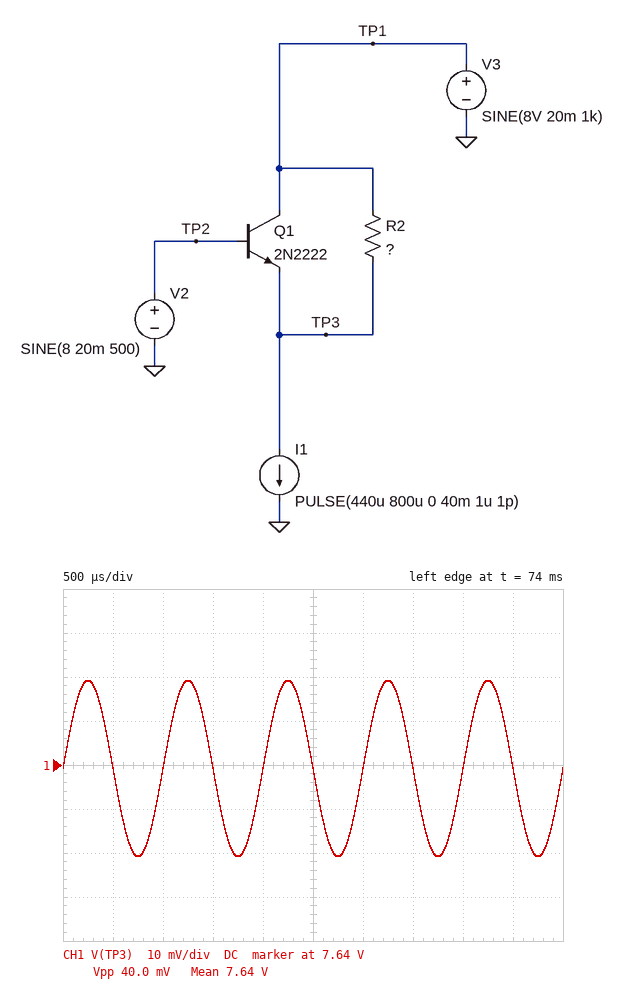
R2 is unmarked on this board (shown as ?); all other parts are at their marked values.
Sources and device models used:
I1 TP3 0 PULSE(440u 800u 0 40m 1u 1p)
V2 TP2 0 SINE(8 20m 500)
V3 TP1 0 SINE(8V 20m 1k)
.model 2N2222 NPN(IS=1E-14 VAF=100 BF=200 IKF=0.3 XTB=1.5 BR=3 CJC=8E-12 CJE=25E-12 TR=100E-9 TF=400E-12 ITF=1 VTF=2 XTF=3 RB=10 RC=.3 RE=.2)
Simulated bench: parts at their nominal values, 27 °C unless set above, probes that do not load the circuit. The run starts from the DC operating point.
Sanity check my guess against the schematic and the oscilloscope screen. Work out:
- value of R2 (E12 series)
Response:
820 Ω
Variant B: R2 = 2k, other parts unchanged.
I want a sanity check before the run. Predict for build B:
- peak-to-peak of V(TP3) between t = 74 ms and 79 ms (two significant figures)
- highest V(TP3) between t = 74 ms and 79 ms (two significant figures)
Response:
37 mV
7.4 V
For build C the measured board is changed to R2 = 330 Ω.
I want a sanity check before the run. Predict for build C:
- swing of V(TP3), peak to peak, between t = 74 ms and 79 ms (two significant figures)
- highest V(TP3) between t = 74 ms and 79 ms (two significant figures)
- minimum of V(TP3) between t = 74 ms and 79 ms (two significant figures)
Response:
40 mV
7.9 V
7.8 V
